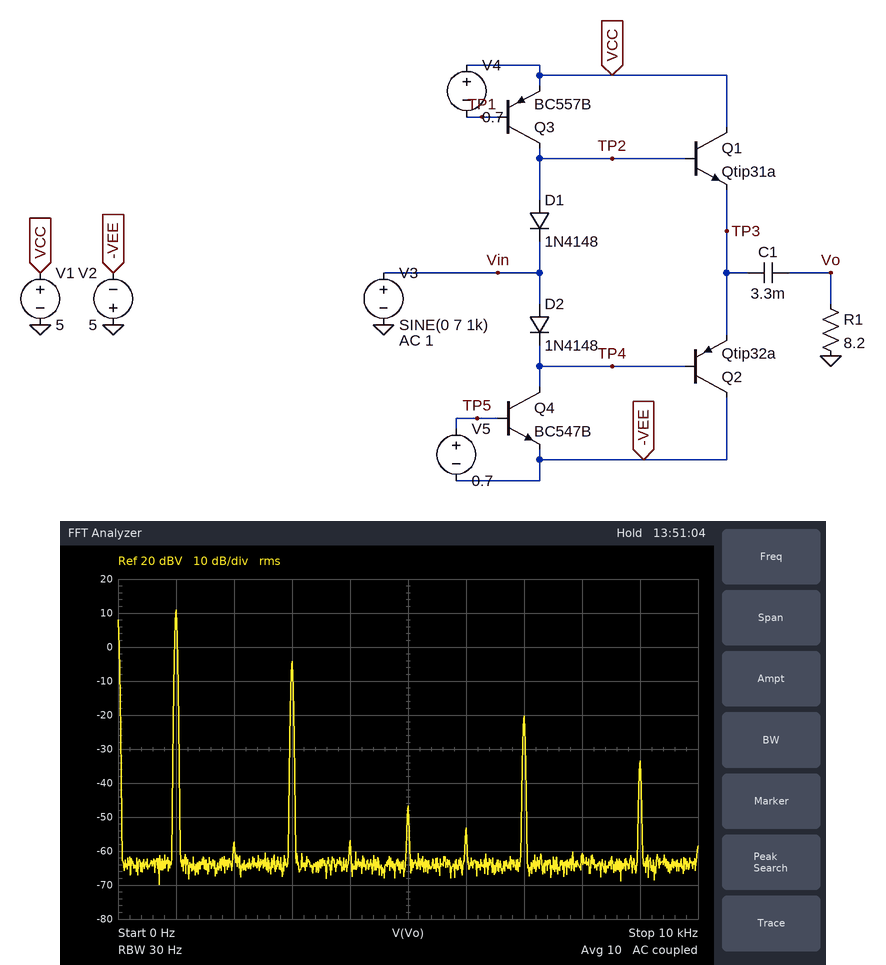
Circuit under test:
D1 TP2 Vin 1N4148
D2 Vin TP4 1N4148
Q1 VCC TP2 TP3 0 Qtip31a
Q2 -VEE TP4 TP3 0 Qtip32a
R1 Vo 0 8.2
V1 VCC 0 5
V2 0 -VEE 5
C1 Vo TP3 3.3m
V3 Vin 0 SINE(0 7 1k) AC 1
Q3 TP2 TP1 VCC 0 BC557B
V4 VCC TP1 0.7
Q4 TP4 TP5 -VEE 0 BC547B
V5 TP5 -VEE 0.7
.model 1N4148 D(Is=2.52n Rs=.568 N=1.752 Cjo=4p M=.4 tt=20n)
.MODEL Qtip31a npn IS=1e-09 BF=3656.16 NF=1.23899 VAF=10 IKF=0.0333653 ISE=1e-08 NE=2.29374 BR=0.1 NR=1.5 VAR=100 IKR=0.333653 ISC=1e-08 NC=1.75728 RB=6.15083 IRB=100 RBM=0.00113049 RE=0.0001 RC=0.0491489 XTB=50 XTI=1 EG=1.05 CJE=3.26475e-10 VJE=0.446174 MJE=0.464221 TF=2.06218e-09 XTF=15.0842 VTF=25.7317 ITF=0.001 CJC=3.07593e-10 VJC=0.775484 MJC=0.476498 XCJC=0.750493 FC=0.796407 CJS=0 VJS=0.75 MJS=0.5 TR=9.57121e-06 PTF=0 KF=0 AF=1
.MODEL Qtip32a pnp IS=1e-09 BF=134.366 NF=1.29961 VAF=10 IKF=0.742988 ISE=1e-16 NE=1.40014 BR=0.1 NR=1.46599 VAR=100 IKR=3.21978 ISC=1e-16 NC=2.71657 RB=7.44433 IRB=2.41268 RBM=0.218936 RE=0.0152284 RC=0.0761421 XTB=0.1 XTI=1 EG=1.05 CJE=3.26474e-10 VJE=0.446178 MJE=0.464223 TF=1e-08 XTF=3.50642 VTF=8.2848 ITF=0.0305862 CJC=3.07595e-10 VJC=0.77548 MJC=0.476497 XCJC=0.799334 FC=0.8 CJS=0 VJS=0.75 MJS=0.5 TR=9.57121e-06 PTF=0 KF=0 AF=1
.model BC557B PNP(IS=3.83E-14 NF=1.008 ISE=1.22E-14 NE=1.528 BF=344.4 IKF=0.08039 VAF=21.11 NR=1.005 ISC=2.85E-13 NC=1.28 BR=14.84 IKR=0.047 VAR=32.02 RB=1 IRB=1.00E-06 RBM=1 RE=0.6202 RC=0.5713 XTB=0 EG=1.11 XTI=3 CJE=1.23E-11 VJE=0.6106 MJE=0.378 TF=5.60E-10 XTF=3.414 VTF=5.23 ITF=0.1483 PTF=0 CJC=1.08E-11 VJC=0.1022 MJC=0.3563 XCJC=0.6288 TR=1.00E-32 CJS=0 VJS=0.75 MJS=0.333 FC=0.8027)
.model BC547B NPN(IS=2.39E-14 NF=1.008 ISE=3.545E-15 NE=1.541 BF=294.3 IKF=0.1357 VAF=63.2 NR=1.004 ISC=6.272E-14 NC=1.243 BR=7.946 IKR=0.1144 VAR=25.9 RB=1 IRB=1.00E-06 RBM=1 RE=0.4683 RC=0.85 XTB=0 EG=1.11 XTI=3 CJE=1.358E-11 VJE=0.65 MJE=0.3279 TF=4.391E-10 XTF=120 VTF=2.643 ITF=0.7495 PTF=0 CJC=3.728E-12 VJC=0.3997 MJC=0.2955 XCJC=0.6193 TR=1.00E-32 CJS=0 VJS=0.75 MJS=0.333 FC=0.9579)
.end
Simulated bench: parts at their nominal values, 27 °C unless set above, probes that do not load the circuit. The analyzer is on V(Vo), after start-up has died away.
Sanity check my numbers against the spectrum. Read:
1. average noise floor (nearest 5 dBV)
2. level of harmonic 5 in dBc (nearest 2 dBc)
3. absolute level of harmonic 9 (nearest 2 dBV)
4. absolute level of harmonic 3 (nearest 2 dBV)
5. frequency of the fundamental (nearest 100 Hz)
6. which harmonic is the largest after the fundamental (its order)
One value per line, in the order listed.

-65 dBV
-58 dBc
-34 dBV
-4 dBV
1.0 kHz
3
